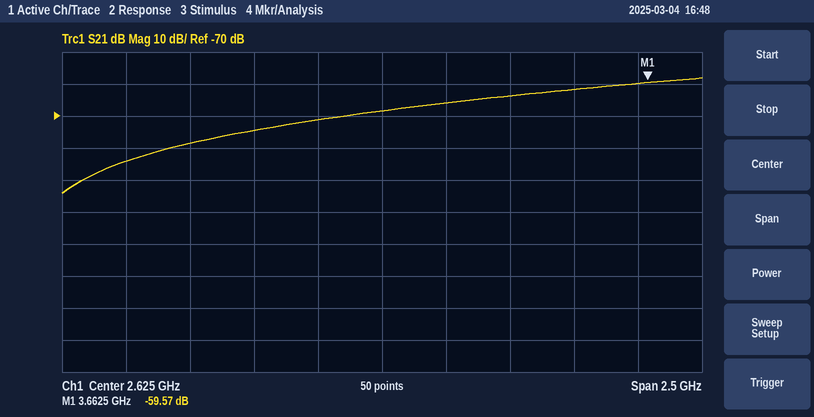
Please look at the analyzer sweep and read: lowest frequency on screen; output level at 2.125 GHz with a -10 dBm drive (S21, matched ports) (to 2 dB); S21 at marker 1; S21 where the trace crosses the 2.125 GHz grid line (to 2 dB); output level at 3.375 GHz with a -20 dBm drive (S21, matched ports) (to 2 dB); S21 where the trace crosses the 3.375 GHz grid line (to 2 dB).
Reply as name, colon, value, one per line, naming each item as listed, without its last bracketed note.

lowest frequency on screen: 1.375 GHz
output level at 2.125 GHz with a -10 dBm drive (S21, matched ports): -84 dBm
S21 at marker 1: -59.57 dB
S21 where the trace crosses the 2.125 GHz grid line: -74 dB
output level at 3.375 GHz with a -20 dBm drive (S21, matched ports): -82 dBm
S21 where the trace crosses the 3.375 GHz grid line: -62 dB
